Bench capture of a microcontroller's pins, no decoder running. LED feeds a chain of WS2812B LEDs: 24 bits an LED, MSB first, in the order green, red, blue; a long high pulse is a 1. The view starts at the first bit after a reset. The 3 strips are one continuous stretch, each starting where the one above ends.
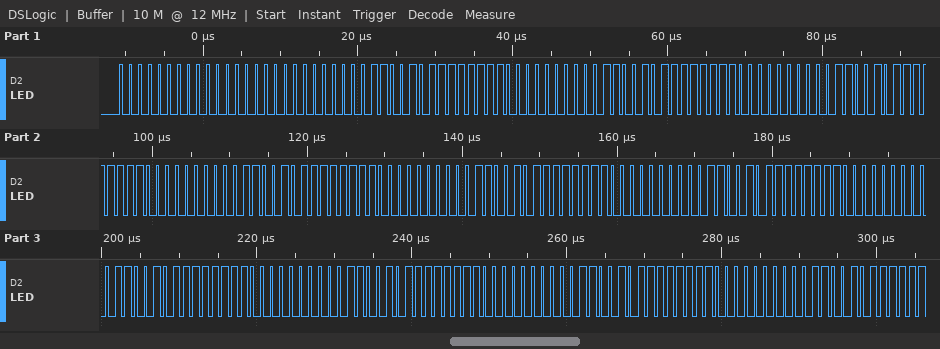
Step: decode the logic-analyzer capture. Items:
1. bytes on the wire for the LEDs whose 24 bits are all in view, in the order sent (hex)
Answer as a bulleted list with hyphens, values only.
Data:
- 00 00 00 32 FF 00 32 FF 00 32 FF 00 32 FF 00 32 FF 00 32 FF 00 32 FF 00 32 FF 00 32 FF 00
